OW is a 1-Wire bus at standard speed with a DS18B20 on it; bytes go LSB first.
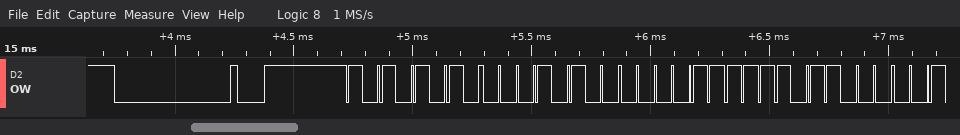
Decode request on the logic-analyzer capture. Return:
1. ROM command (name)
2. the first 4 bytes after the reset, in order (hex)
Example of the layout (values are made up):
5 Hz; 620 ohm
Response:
Match ROM; 55 28 F0 1B
